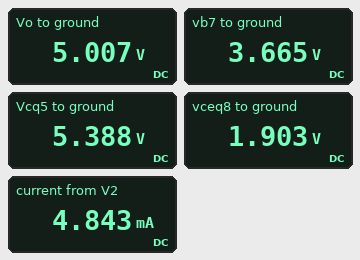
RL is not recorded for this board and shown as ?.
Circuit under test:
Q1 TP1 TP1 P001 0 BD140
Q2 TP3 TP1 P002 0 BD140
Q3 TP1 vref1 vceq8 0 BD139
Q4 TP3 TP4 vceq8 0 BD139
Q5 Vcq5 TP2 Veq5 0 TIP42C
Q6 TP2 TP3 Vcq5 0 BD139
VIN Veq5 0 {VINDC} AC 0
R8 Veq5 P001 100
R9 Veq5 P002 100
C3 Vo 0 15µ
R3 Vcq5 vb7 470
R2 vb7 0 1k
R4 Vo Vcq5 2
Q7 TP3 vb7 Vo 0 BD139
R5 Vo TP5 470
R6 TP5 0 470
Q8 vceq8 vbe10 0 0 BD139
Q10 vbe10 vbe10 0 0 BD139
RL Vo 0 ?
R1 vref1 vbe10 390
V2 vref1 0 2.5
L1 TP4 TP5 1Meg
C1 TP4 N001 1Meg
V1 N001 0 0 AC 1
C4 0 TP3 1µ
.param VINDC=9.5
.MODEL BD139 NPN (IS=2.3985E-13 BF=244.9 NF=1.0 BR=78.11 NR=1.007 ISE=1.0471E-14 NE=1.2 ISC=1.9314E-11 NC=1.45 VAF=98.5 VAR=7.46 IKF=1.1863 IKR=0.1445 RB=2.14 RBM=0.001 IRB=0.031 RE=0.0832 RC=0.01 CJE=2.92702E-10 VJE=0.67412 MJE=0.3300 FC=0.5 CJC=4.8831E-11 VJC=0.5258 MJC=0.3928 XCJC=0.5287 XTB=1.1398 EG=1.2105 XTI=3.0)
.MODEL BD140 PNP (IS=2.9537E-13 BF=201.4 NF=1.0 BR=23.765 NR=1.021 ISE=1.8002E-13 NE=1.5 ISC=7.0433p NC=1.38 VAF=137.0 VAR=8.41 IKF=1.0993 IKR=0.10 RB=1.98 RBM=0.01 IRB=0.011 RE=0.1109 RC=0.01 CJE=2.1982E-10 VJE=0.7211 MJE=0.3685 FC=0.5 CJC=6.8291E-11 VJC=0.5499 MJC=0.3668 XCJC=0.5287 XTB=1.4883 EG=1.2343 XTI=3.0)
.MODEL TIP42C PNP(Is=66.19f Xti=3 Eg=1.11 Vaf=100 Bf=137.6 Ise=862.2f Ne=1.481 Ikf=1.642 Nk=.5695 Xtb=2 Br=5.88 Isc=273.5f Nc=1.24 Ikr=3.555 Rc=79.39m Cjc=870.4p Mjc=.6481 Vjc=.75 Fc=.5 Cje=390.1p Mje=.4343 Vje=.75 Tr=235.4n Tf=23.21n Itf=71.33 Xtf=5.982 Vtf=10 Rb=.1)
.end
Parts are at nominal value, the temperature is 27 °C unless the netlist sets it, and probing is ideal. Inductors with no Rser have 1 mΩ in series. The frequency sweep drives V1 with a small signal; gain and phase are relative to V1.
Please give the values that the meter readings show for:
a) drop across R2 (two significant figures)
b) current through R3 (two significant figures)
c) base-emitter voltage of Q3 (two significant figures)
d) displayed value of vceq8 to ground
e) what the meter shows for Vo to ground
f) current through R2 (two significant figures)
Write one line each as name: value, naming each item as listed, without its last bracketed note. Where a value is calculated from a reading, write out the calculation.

drop across R2: 3.665 V = 3.7 V
current through R3: (5.388 V - 3.665 V) / 470 Ω = 3.7 mA
base-emitter voltage of Q3: 2.5 V - 1.903 V = 600 mV
displayed value of vceq8 to ground: 1.903 V
what the meter shows for Vo to ground: 5.007 V
current through R2: (3.665 V) / 1 kΩ = 3.7 mA
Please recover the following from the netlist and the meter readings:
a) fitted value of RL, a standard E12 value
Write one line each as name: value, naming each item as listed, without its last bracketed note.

fitted value of RL, a standard E12 value: 27 Ω
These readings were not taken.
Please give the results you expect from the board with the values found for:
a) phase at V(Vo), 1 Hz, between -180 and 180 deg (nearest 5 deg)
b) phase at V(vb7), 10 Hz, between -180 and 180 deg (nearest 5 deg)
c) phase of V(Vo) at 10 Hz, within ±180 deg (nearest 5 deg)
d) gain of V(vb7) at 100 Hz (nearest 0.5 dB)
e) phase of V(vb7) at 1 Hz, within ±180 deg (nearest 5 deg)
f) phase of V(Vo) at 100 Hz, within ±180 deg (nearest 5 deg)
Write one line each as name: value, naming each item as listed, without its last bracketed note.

phase at V(Vo), 1 Hz, between -180 and 180 deg: 170 deg
phase at V(vb7), 10 Hz, between -180 and 180 deg: 115 deg
phase of V(Vo) at 10 Hz, within ±180 deg: 115 deg
gain of V(vb7) at 100 Hz: 40.0 dB
phase of V(vb7) at 1 Hz, within ±180 deg: 170 deg
phase of V(Vo) at 100 Hz, within ±180 deg: 90 deg
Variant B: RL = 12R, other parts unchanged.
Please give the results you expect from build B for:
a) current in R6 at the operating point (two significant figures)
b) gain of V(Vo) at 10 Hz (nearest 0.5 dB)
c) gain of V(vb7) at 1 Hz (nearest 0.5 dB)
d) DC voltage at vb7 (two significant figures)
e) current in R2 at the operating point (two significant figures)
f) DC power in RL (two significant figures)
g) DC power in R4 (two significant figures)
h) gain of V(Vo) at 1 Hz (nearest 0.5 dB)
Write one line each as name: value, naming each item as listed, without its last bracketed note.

current in R6 at the operating point: 5.3 mA
gain of V(Vo) at 10 Hz: 61.0 dB
gain of V(vb7) at 1 Hz: 65.5 dB
DC voltage at vb7: 4.0 V
current in R2 at the operating point: 4.0 mA
DC power in RL: 2.1 W
DC power in R4: 360 mW
gain of V(Vo) at 1 Hz: 67.5 dB
